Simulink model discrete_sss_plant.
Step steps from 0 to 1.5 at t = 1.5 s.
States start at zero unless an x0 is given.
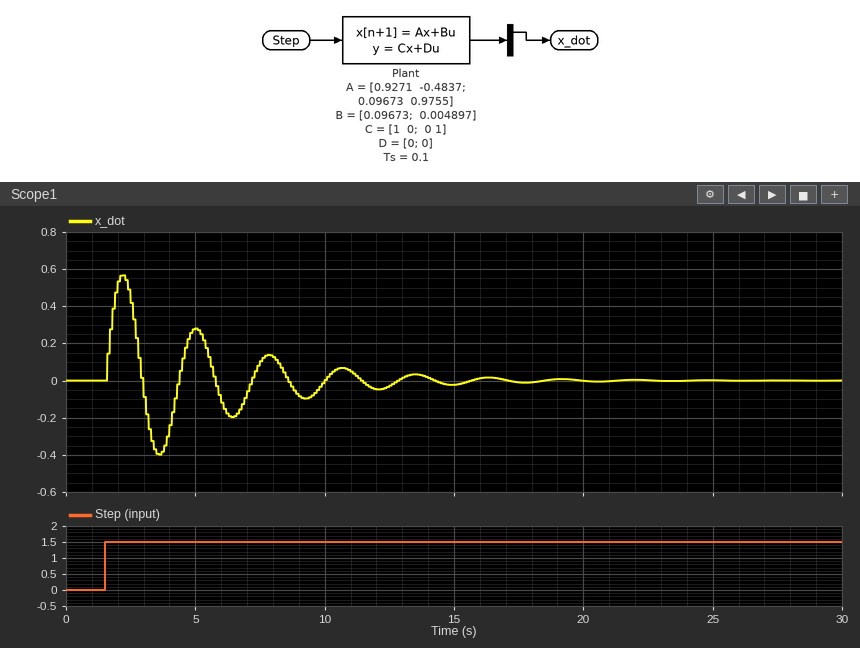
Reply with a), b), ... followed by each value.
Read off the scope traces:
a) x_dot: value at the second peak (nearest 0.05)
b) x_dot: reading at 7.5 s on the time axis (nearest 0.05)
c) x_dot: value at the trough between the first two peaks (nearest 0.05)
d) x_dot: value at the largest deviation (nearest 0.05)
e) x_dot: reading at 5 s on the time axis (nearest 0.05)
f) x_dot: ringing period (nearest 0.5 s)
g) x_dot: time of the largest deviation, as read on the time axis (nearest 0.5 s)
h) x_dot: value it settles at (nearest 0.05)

a) 0.30
b) 0.10
c) -0.40
d) 0.55
e) 0.30
f) 3.0 s
g) 2.0 s
h) 0.00
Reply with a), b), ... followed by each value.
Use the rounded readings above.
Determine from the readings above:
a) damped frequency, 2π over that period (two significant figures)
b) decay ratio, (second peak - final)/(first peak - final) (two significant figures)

a) 2.1 rad/s
b) 0.55
